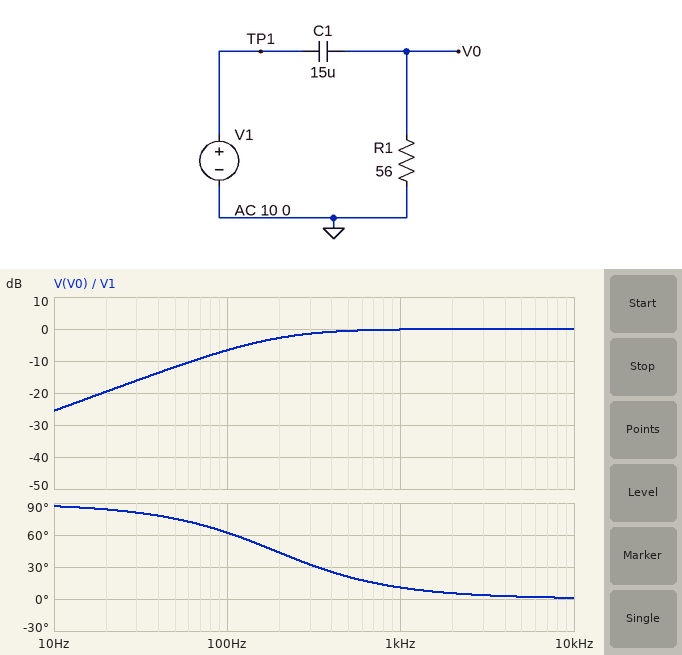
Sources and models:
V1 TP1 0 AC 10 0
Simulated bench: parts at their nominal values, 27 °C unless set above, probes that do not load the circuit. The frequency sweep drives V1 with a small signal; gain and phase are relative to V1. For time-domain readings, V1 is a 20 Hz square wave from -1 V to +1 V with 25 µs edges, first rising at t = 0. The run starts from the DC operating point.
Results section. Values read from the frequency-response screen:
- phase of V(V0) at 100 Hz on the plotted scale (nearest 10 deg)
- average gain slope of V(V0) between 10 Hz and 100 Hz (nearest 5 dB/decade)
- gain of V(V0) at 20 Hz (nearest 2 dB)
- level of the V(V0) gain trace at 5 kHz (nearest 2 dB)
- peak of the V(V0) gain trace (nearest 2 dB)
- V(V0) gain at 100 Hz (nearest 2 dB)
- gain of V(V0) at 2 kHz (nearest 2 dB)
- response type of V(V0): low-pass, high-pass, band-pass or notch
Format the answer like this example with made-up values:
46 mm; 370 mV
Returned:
60 deg; 20 dB/decade; -20 dB; 0 dB; 0 dB; -6 dB; 0 dB; high-pass
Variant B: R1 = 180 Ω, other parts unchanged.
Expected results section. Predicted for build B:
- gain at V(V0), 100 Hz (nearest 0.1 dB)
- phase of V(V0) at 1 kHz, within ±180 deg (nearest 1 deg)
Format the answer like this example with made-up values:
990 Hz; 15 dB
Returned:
-1.3 dB; 3 deg
